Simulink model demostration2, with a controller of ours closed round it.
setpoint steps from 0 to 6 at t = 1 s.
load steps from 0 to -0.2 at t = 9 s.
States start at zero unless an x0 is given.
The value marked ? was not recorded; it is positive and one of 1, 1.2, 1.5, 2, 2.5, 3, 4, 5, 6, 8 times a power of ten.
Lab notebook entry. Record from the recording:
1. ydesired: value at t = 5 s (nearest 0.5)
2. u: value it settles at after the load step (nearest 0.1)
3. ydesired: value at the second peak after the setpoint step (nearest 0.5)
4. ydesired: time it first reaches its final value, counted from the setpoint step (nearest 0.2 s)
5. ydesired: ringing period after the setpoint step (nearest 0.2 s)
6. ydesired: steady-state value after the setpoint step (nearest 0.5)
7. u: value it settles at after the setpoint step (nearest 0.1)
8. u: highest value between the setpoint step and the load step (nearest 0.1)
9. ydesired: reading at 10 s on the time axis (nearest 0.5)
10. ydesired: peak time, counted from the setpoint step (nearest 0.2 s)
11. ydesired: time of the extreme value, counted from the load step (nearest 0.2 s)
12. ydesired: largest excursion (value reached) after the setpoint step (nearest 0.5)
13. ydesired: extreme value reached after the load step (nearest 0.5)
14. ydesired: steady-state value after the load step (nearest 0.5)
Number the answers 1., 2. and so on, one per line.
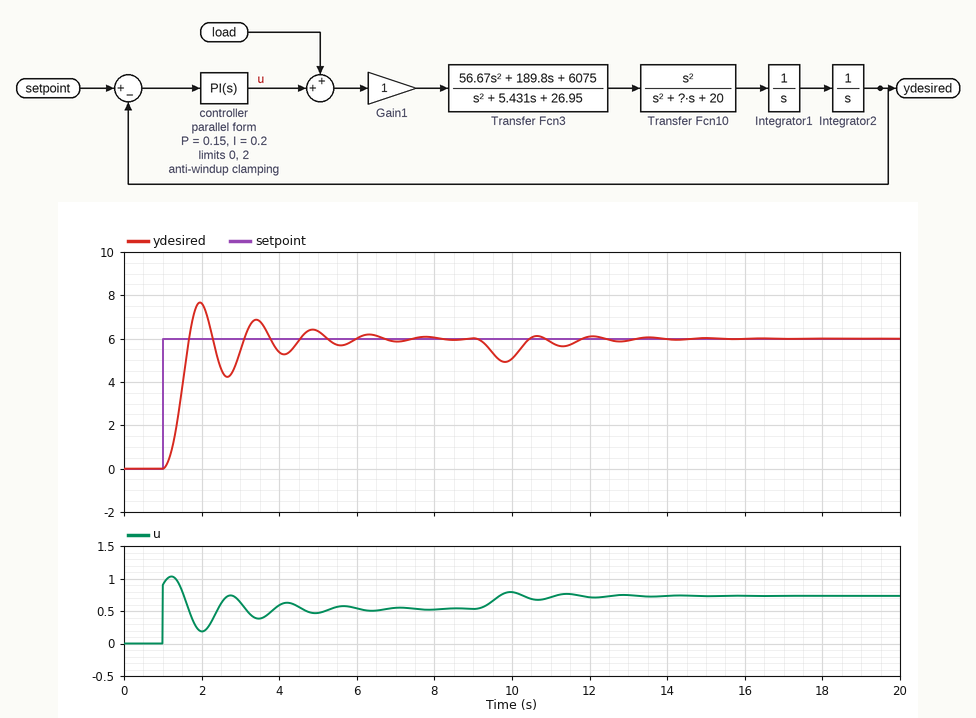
1. 6.5
2. 0.7
3. 7.0
4. 0.6 s
5. 1.4 s
6. 6.0
7. 0.5
8. 1.0
9. 5.0
10. 1.0 s
11. 0.8 s
12. 7.5
13. 5.0
14. 6.0
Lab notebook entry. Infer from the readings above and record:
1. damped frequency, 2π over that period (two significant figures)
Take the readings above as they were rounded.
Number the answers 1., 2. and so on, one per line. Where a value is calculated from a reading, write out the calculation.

1. 2π / 1.4 = 4.5 rad/s
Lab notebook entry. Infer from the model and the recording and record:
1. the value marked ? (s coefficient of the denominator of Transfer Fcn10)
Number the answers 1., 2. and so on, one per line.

1. 10
